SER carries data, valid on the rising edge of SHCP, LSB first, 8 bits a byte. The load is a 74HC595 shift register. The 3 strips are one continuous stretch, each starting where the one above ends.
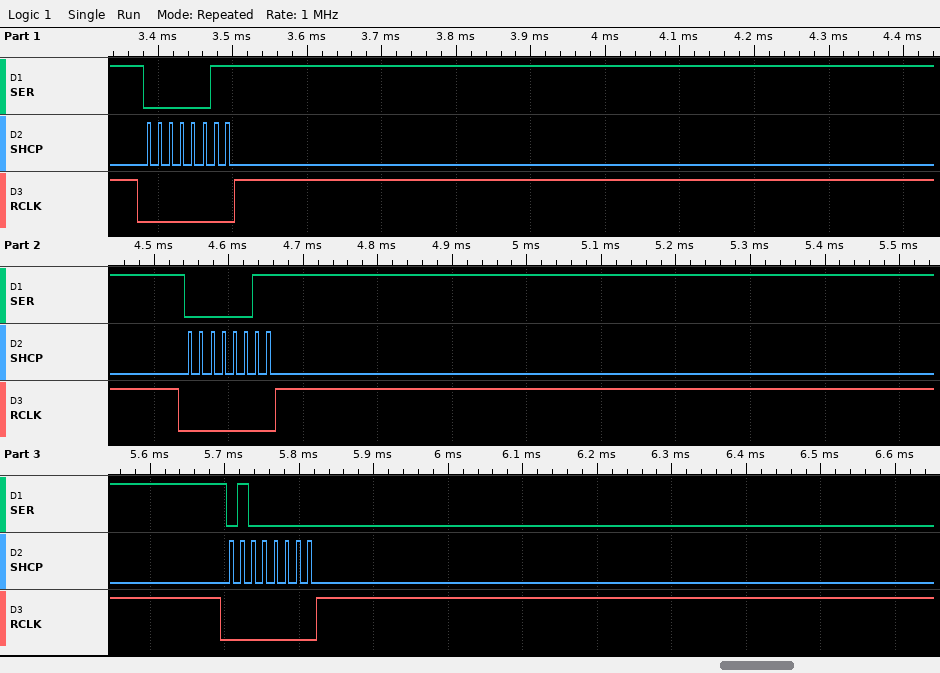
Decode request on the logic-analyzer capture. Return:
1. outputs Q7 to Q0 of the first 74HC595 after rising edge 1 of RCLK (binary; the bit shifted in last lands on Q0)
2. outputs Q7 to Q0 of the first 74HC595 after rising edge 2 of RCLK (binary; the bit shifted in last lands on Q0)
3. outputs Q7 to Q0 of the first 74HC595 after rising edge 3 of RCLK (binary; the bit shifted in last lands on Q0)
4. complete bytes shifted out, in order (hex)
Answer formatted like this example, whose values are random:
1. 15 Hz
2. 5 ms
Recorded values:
1. 00000011
2. 00000011
3. 01000000
4. C0 C0 02
